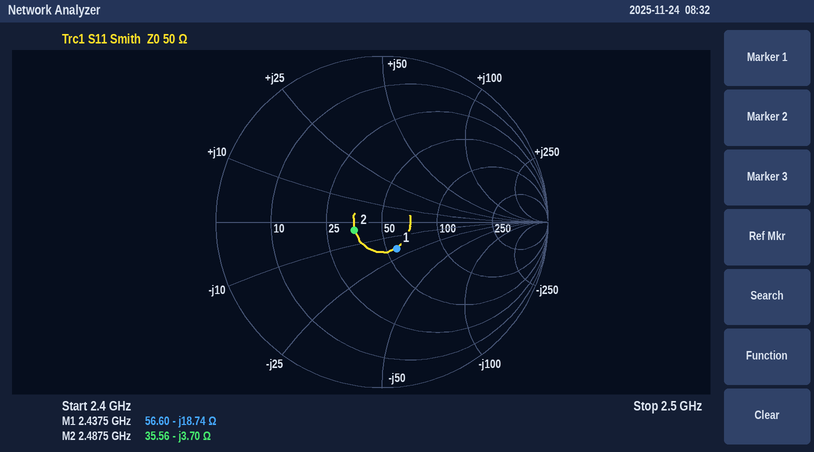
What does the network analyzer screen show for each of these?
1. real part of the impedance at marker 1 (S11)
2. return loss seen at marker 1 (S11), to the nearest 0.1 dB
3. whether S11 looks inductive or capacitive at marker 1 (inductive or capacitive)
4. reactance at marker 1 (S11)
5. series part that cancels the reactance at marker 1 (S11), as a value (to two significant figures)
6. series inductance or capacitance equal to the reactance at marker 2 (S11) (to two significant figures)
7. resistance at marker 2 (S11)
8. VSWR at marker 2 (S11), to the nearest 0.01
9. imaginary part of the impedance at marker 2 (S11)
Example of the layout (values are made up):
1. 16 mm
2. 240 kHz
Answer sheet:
1. 56.60 Ω
2. 14.7 dB
3. capacitive
4. -18.74 Ω
5. 1.2 nH
6. 17 pF
7. 35.56 Ω
8. 1.42
9. -3.70 Ω
